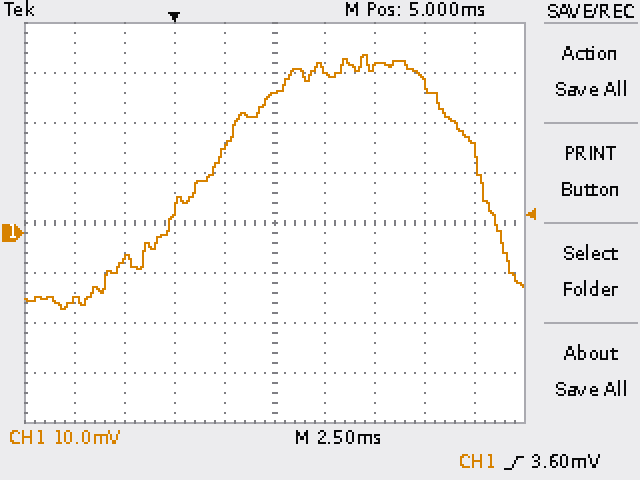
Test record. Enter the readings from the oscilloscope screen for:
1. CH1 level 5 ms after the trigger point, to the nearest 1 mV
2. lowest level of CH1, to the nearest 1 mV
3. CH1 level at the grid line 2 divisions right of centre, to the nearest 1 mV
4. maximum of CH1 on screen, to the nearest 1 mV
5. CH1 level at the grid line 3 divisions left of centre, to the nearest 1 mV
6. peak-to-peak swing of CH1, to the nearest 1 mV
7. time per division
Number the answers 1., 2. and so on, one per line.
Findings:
1. 28 mV
2. -15 mV
3. 33 mV
4. 36 mV
5. -5 mV
6. 51 mV
7. 2.5 ms
